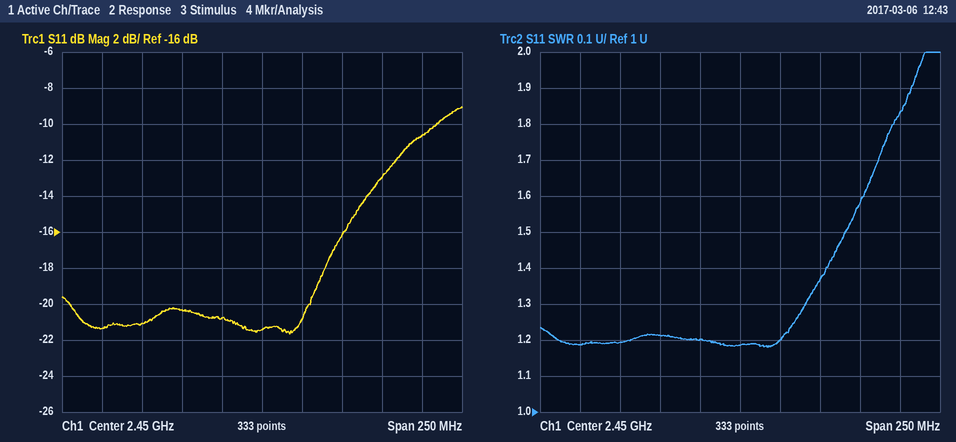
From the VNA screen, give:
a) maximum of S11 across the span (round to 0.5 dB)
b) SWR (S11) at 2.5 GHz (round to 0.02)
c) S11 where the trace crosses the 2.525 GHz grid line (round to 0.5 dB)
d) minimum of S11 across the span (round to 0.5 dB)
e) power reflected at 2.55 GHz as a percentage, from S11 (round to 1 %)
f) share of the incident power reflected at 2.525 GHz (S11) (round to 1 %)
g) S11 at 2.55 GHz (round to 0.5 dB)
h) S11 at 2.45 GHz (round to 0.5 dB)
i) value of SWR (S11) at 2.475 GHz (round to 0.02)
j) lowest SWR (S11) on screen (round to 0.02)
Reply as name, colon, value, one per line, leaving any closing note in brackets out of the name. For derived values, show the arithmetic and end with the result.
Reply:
maximum of S11 across the span: -9.0 dB
SWR (S11) at 2.5 GHz: 1.36
S11 where the trace crosses the 2.525 GHz grid line: -13.0 dB
minimum of S11 across the span: -21.5 dB
power reflected at 2.55 GHz as a percentage, from S11: 10^(-10.5/10) ≈ 9 %
share of the incident power reflected at 2.525 GHz (S11): 10^(-13/10) ≈ 5 %
S11 at 2.55 GHz: -10.5 dB
S11 at 2.45 GHz: -21.5 dB
value of SWR (S11) at 2.475 GHz: 1.20
lowest SWR (S11) on screen: 1.18
